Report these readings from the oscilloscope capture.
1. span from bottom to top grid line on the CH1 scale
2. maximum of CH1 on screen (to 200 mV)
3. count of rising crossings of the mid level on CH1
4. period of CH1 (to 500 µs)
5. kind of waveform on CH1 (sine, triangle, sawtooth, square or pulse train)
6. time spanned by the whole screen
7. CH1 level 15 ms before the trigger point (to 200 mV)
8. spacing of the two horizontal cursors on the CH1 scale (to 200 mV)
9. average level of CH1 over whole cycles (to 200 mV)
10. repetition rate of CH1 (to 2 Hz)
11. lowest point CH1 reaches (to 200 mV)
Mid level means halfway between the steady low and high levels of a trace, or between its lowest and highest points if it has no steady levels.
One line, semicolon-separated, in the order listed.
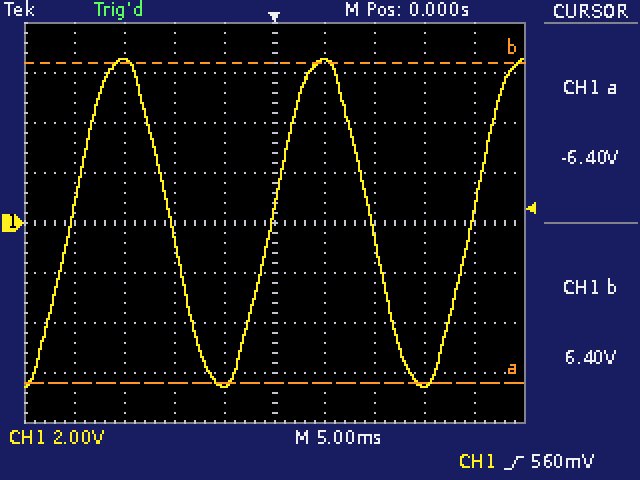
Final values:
16 V; 6.6 V; 3; 20.0 ms; sine; 50 ms; 6.6 V; 12.8 V; 0.0 V; 50 Hz; -6.6 V
